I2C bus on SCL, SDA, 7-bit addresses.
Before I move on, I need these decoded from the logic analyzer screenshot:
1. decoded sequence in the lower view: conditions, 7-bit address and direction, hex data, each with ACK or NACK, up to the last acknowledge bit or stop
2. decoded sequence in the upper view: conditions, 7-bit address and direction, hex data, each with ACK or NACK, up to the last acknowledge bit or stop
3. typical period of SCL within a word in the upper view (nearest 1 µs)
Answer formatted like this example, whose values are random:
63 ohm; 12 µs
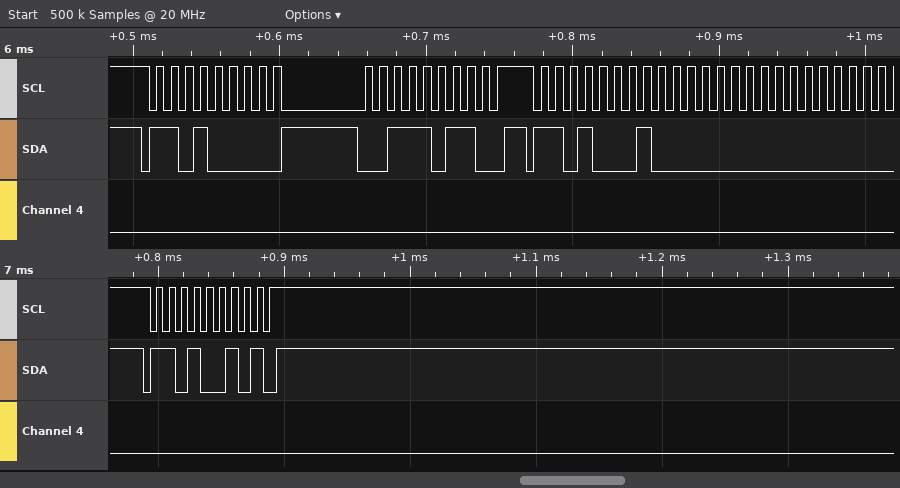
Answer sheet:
start, address 69 write NACK, stop; start, address 68 write ACK, 3B ACK, stop, start, address 68 read ACK, 00 ACK; 10 µs
